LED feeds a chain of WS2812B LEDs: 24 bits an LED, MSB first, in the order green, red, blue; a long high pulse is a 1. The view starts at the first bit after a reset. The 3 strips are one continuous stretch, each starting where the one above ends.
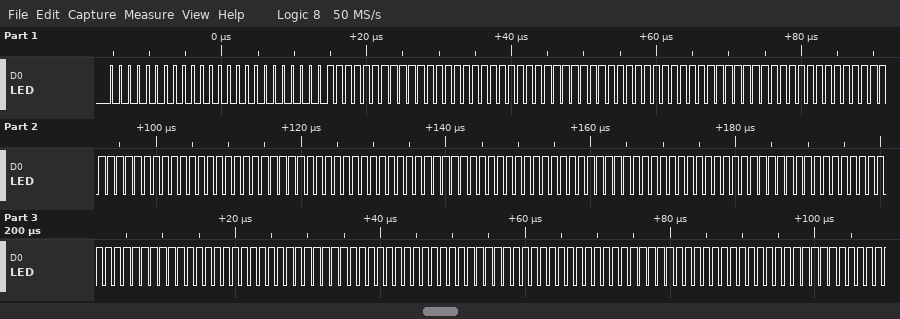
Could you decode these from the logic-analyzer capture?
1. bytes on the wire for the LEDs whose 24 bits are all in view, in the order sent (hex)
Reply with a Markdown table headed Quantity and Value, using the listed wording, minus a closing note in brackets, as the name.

| Quantity | Value |
|---|---|
| bytes on the wire for the LEDs whose 24 bits are all in view, in the order sent | 00 00 00 FF FF FF FF FF FF FF FF FF FF FF FF FF FF FF FF FF FF FF FF FF FF FF FF FF FF FF |
